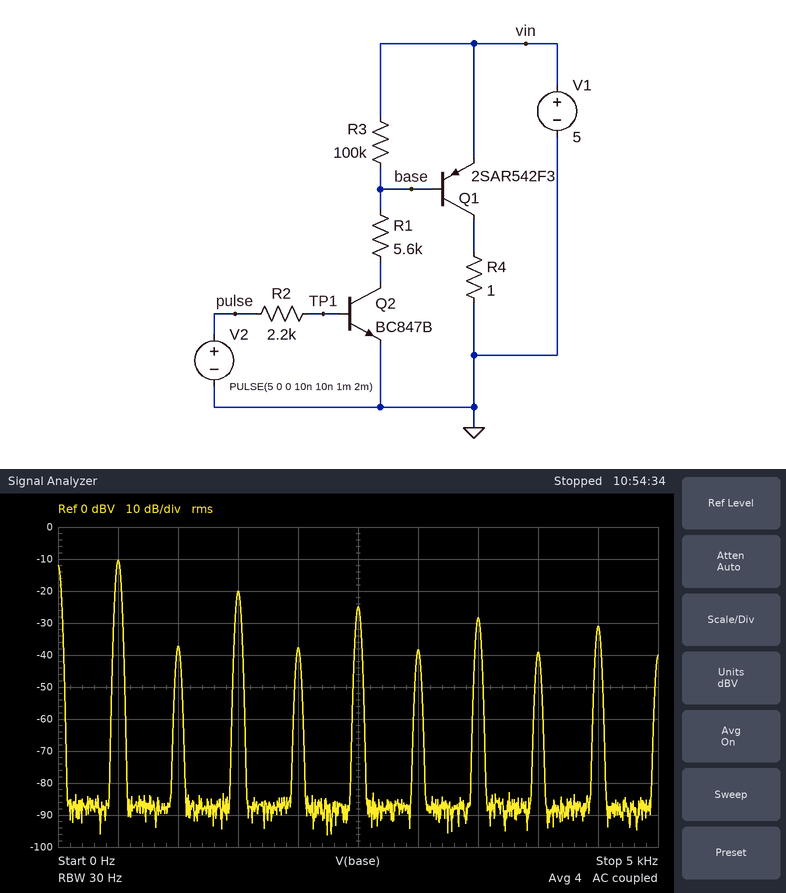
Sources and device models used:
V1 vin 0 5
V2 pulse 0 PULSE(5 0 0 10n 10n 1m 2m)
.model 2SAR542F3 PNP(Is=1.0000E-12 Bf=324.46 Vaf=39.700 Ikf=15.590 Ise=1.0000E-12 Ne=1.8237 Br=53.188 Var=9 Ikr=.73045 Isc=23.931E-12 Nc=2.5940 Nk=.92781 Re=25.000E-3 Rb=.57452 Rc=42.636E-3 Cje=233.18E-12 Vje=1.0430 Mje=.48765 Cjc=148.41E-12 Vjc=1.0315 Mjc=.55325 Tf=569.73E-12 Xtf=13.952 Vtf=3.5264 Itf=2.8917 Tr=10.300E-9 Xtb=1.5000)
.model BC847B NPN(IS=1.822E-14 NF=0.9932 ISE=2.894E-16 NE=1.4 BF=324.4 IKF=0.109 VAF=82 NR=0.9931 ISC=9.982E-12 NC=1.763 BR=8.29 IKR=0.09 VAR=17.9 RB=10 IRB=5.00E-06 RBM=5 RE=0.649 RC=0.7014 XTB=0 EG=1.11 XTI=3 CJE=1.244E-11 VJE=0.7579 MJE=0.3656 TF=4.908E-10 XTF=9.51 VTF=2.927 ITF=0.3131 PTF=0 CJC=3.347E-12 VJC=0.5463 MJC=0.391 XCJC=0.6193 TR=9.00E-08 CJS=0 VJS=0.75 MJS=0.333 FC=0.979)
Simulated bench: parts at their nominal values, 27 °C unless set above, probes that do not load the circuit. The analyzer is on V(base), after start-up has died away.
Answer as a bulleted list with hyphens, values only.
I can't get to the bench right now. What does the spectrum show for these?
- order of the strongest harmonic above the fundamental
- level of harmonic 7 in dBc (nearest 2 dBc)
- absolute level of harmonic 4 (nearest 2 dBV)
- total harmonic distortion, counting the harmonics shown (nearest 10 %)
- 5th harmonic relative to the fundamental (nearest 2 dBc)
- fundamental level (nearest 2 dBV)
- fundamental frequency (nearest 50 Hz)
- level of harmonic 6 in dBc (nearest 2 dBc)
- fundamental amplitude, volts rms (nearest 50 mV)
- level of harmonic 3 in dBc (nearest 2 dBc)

- 3
- -18 dBc
- -38 dBV
- 40 %
- -14 dBc
- -10 dBV
- 500 Hz
- -28 dBc
- 300 mV
- -10 dBc
